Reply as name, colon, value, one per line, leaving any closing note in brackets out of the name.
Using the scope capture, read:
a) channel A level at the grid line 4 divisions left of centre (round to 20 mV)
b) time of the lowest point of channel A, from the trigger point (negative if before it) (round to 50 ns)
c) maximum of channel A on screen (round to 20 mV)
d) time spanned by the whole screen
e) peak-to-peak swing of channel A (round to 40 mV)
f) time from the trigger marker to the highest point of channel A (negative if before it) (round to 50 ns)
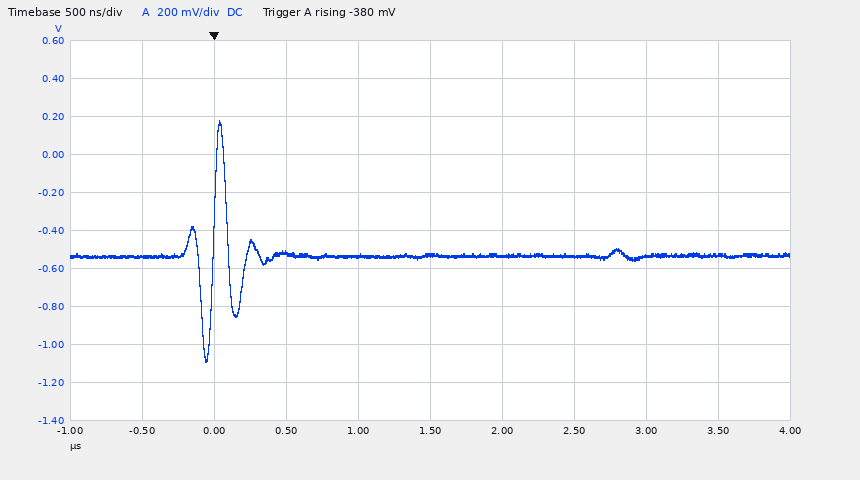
channel A level at the grid line 4 divisions left of centre: -540 mV
time of the lowest point of channel A, from the trigger point (negative if before it): -50 ns
maximum of channel A on screen: 180 mV
time spanned by the whole screen: 5 µs
peak-to-peak swing of channel A: 1.28 V
time from the trigger marker to the highest point of channel A (negative if before it): +50 ns
